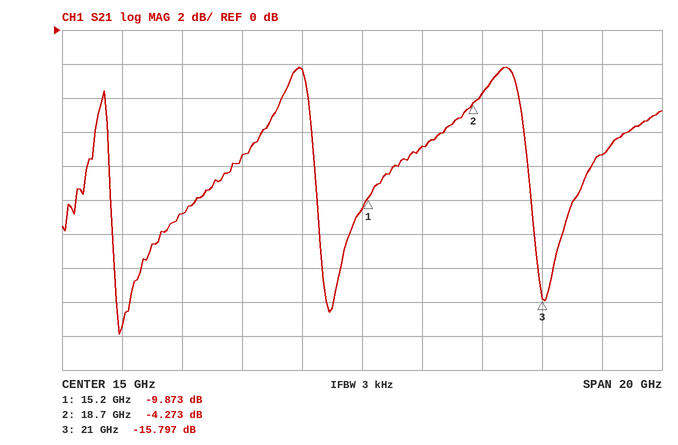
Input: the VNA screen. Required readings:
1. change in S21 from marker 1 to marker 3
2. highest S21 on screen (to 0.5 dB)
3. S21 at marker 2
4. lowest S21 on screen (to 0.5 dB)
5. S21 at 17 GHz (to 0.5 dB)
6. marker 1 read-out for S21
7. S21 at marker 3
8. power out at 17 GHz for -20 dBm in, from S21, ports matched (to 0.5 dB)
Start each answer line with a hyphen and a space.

- -5.924 dB
- -2.0 dB
- -4.273 dB
- -18.0 dB
- -7.0 dB
- -9.873 dB
- -15.797 dB
- -27.0 dBm
